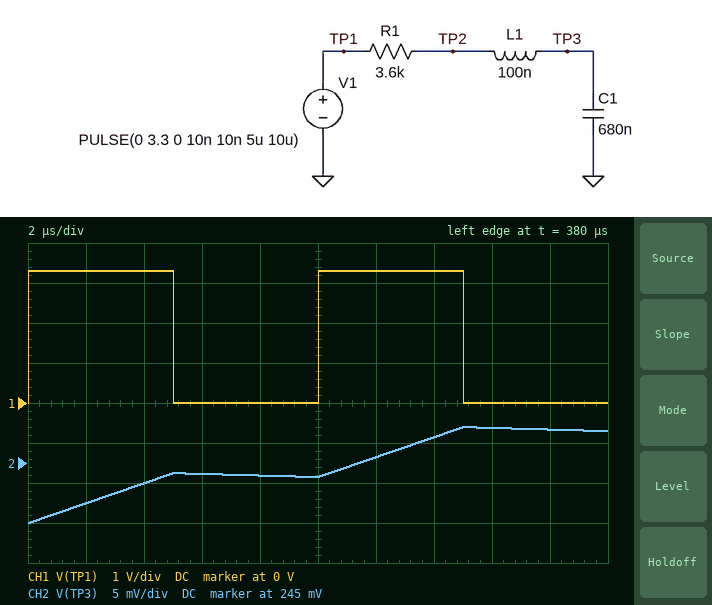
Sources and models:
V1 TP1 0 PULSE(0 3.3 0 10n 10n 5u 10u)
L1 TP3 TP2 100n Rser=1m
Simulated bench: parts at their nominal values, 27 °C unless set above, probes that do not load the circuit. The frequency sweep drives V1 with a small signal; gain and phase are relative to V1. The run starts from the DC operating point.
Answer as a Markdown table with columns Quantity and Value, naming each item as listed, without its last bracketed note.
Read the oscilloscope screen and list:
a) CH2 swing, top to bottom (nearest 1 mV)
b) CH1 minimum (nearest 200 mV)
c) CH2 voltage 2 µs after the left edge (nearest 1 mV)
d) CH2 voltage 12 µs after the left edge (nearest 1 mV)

| Quantity | Value |
|---|---|
| CH2 swing, top to bottom | 12 mV |
| CH1 minimum | 0 V |
| CH2 voltage 2 µs after the left edge | 240 mV |
| CH2 voltage 12 µs after the left edge | 246 mV |
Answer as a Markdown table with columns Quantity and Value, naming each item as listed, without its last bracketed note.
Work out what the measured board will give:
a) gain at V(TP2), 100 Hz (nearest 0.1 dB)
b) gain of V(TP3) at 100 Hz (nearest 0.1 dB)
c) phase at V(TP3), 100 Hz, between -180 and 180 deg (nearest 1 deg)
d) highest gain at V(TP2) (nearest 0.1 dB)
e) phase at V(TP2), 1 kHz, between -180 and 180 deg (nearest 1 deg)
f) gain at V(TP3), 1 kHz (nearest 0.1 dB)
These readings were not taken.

| Quantity | Value |
|---|---|
| gain at V(TP2), 100 Hz | -5.3 dB |
| gain of V(TP3) at 100 Hz | -5.3 dB |
| phase at V(TP3), 100 Hz, between -180 and 180 deg | -57 deg |
| highest gain at V(TP2) | 0 dB |
| phase at V(TP2), 1 kHz, between -180 and 180 deg | -86 deg |
| gain at V(TP3), 1 kHz | -23.8 dB |
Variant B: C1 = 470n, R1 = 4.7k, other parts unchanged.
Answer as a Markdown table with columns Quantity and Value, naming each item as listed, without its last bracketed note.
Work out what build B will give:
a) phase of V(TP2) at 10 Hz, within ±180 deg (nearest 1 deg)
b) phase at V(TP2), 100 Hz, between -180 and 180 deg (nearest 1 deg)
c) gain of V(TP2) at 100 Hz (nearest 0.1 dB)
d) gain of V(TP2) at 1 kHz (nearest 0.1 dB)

| Quantity | Value |
|---|---|
| phase of V(TP2) at 10 Hz, within ±180 deg | -8 deg |
| phase at V(TP2), 100 Hz, between -180 and 180 deg | -54 deg |
| gain of V(TP2) at 100 Hz | -4.7 dB |
| gain of V(TP2) at 1 kHz | -22.9 dB |
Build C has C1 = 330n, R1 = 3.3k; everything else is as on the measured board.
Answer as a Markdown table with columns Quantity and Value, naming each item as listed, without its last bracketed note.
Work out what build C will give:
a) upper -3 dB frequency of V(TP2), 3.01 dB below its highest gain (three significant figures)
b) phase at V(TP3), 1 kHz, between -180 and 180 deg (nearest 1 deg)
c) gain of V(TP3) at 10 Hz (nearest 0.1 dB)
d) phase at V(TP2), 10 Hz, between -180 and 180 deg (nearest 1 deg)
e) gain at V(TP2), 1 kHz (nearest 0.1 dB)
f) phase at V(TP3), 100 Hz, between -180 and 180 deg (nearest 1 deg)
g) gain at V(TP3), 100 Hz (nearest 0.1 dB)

| Quantity | Value |
|---|---|
| upper -3 dB frequency of V(TP2), 3.01 dB below its highest gain | 146 Hz |
| phase at V(TP3), 1 kHz, between -180 and 180 deg | -82 deg |
| gain of V(TP3) at 10 Hz | 0 dB |
| phase at V(TP2), 10 Hz, between -180 and 180 deg | -4 deg |
| gain at V(TP2), 1 kHz | -16.8 dB |
| phase at V(TP3), 100 Hz, between -180 and 180 deg | -34 deg |
| gain at V(TP3), 100 Hz | -1.7 dB |
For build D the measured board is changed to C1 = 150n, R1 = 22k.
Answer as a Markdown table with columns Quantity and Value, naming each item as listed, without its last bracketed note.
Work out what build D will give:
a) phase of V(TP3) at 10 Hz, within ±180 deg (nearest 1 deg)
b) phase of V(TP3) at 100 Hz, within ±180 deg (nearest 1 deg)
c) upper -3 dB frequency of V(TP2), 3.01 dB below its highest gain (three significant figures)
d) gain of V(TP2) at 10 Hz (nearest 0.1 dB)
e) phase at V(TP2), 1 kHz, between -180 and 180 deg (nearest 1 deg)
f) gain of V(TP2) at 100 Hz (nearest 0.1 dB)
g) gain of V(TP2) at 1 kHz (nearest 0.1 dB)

| Quantity | Value |
|---|---|
| phase of V(TP3) at 10 Hz, within ±180 deg | -12 deg |
| phase of V(TP3) at 100 Hz, within ±180 deg | -64 deg |
| upper -3 dB frequency of V(TP2), 3.01 dB below its highest gain | 48.2 Hz |
| gain of V(TP2) at 10 Hz | -0.2 dB |
| phase at V(TP2), 1 kHz, between -180 and 180 deg | -87 deg |
| gain of V(TP2) at 100 Hz | -7.2 dB |
| gain of V(TP2) at 1 kHz | -26.3 dB |
